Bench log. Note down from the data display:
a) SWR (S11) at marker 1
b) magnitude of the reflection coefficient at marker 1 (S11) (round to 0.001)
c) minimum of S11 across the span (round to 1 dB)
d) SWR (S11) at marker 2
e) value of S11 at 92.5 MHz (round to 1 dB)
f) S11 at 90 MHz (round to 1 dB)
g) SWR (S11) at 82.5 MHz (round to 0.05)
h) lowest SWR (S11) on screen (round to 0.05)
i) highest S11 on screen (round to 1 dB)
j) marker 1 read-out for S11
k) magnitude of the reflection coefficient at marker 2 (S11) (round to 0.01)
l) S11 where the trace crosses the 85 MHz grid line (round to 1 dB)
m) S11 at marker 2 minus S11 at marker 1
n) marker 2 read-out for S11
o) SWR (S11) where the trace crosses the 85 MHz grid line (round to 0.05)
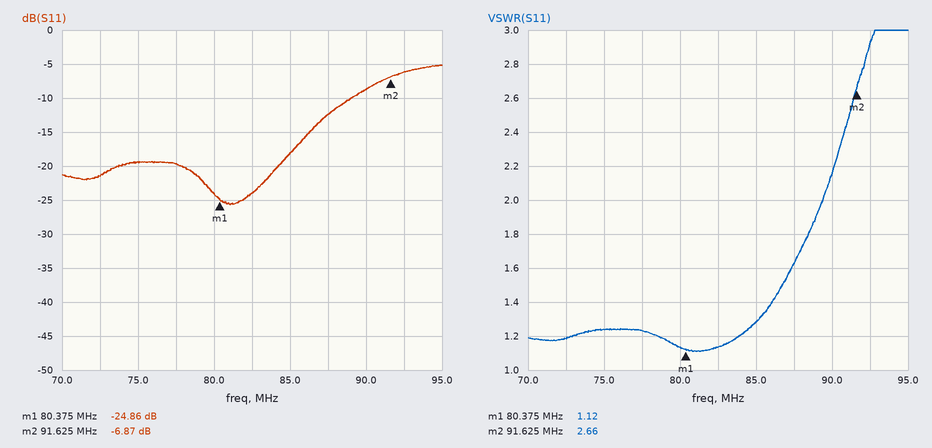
1.12
0.057
-26 dB
2.66
-6 dB
-9 dB
1.15
1.10
-5 dB
-24.86 dB
0.45
-18 dB
17.99 dB
-6.87 dB
1.30
